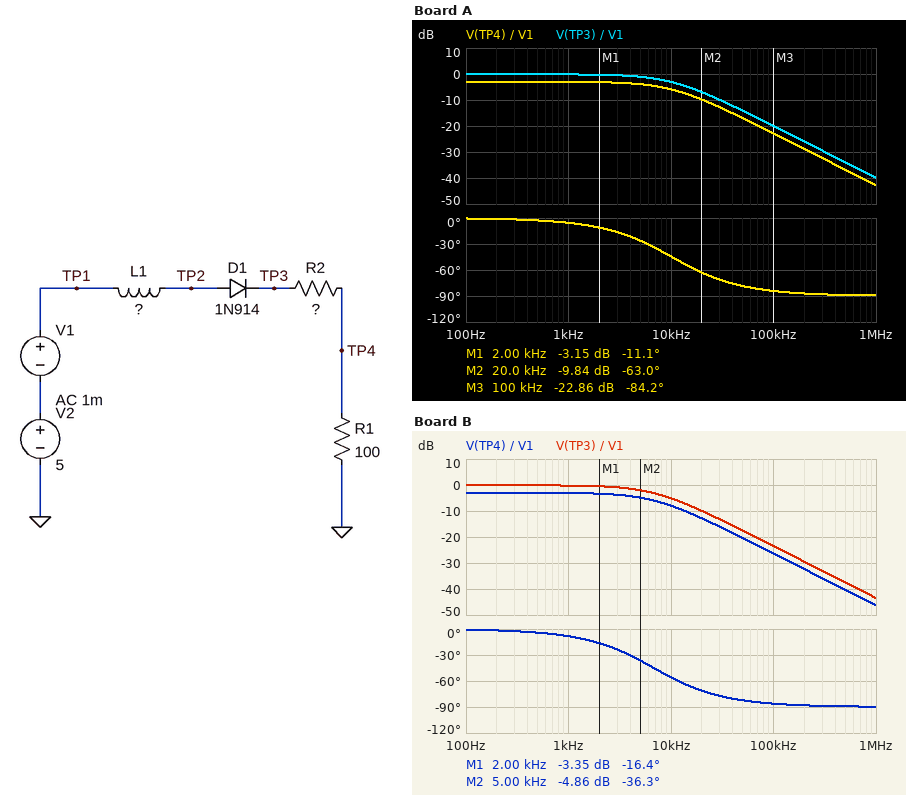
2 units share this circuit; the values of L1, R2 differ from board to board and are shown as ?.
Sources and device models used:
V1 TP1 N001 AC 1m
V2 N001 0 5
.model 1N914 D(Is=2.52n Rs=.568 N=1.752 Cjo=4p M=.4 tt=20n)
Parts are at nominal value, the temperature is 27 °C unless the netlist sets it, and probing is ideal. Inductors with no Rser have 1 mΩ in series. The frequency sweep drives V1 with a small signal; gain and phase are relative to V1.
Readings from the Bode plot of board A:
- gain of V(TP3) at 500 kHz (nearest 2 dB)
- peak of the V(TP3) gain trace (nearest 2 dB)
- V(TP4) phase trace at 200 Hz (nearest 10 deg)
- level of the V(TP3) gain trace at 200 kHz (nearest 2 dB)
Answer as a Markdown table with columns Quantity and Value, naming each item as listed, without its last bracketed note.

| Quantity | Value |
|---|---|
| gain of V(TP3) at 500 kHz | -34 dB |
| peak of the V(TP3) gain trace | 0 dB |
| V(TP4) phase trace at 200 Hz | 0 deg |
| level of the V(TP3) gain trace at 200 kHz | -26 dB |
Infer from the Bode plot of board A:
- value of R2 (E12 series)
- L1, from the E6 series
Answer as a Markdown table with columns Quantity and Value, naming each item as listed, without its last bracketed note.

| Quantity | Value |
|---|---|
| value of R2 | 39 Ω |
| L1, from the E6 series | 2.2 mH |
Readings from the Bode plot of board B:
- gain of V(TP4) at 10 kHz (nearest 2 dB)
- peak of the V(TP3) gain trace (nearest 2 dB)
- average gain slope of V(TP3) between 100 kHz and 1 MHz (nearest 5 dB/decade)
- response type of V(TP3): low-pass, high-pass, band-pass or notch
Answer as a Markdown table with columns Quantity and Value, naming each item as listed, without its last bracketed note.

| Quantity | Value |
|---|---|
| gain of V(TP4) at 10 kHz | -8 dB |
| peak of the V(TP3) gain trace | 0 dB |
| average gain slope of V(TP3) between 100 kHz and 1 MHz | -20 dB/decade |
| response type of V(TP3): low-pass, high-pass, band-pass or notch | low-pass |
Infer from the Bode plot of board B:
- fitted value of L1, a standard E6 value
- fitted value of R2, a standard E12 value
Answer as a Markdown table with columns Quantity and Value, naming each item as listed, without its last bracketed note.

| Quantity | Value |
|---|---|
| fitted value of L1, a standard E6 value | 3.3 mH |
| fitted value of R2, a standard E12 value | 39 Ω |
